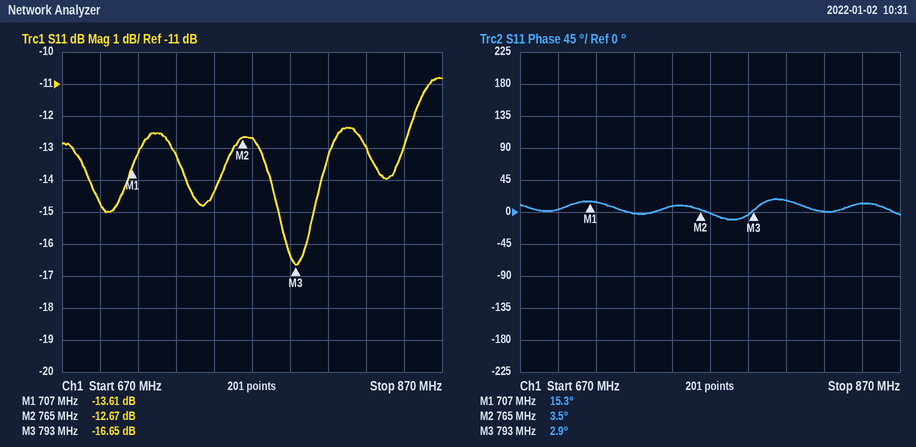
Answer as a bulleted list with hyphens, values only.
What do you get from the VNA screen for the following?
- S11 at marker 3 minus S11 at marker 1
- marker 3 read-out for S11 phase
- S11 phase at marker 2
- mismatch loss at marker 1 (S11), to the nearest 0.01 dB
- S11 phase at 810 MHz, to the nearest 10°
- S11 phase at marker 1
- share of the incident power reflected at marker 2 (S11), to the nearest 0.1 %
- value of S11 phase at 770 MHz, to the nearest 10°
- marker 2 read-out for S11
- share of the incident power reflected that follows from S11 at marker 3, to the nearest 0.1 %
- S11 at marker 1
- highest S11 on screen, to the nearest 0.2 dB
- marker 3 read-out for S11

- -3.04 dB
- 2.9°
- 3.5°
- 0.19 dB
- 20°
- 15.3°
- 5.4 %
- 0°
- -12.67 dB
- 2.2 %
- -13.61 dB
- -10.8 dB
- -16.65 dB
